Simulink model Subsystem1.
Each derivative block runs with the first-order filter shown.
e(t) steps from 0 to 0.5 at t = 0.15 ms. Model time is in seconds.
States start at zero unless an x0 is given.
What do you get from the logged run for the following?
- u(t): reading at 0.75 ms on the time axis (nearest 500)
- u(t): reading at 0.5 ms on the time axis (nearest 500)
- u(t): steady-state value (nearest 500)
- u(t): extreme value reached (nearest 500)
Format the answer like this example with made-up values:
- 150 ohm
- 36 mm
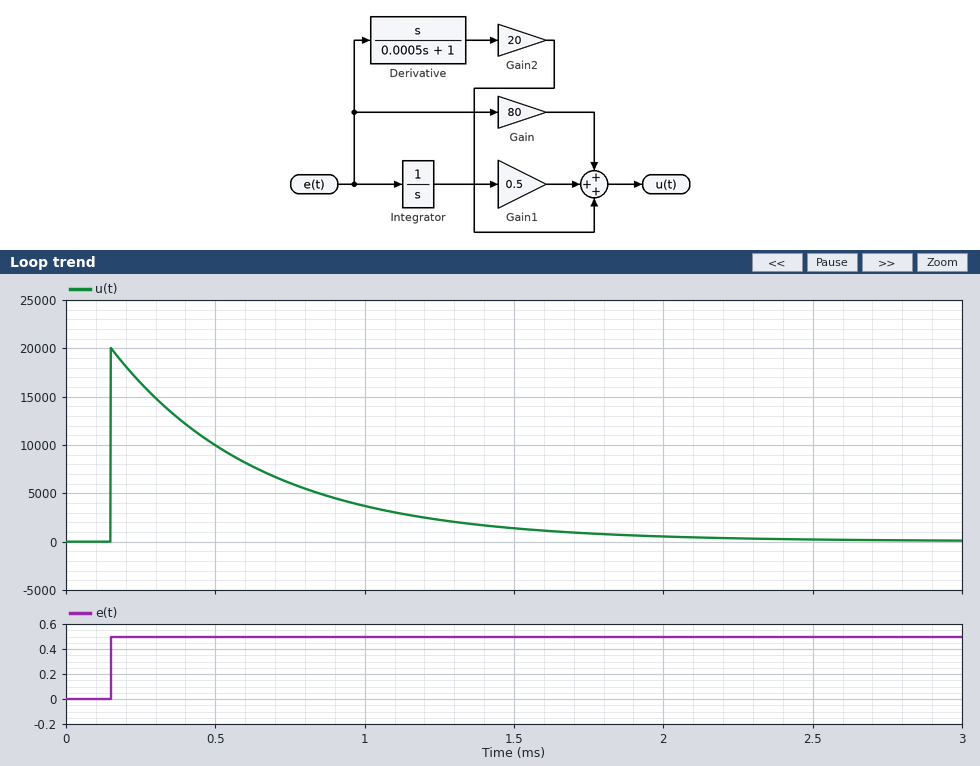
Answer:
- 6000
- 10000
- 0
- 20000
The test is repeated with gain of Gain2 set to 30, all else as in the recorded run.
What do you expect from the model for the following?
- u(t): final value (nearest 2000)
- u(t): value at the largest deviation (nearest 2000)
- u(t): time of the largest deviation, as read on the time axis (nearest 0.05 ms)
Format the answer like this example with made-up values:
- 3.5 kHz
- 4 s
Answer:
- 0
- 30000
- 0.15 ms
